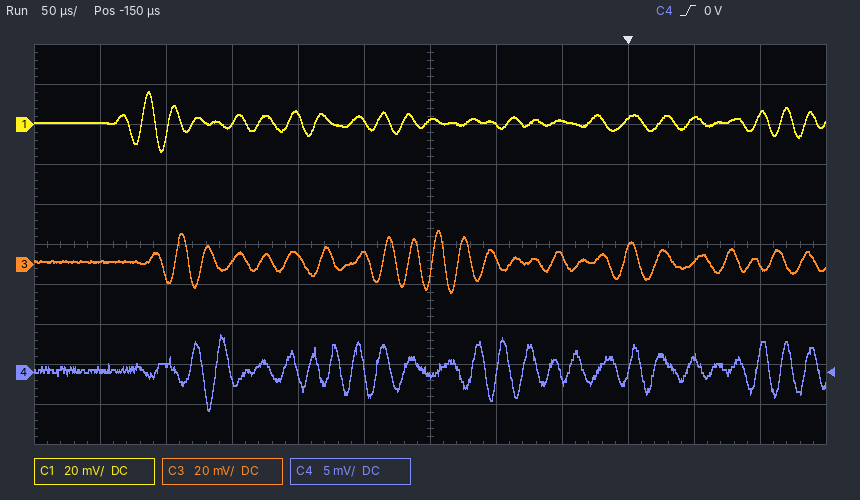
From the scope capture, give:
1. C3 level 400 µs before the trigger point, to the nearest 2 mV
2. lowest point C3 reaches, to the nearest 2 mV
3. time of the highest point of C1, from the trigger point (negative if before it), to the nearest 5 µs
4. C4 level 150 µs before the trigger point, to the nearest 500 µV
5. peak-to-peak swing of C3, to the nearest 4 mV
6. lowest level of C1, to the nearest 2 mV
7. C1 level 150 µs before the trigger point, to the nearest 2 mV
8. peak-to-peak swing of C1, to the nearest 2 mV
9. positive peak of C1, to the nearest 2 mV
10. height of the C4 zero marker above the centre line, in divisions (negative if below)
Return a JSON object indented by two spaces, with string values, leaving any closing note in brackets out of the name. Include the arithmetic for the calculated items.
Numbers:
{
  "C3 level 400 µs before the trigger point, to the nearest 2 mV": "2 mV",
  "lowest point C3 reaches, to the nearest 2 mV": "-14 mV",
  "time of the highest point of C1, from the trigger point (negative if before it), to the nearest 5 µs": "-365 µs",
  "C4 level 150 µs before the trigger point, to the nearest 500 µV": "-500 µV",
  "peak-to-peak swing of C3, to the nearest 4 mV": "32 mV",
  "lowest level of C1, to the nearest 2 mV": "-14 mV",
  "C1 level 150 µs before the trigger point, to the nearest 2 mV": "2 mV",
  "peak-to-peak swing of C1, to the nearest 2 mV": "16 mV − (-14 mV) = 30 mV",
  "positive peak of C1, to the nearest 2 mV": "16 mV",
  "height of the C4 zero marker above the centre line, in divisions": "-3.2 div"
}
